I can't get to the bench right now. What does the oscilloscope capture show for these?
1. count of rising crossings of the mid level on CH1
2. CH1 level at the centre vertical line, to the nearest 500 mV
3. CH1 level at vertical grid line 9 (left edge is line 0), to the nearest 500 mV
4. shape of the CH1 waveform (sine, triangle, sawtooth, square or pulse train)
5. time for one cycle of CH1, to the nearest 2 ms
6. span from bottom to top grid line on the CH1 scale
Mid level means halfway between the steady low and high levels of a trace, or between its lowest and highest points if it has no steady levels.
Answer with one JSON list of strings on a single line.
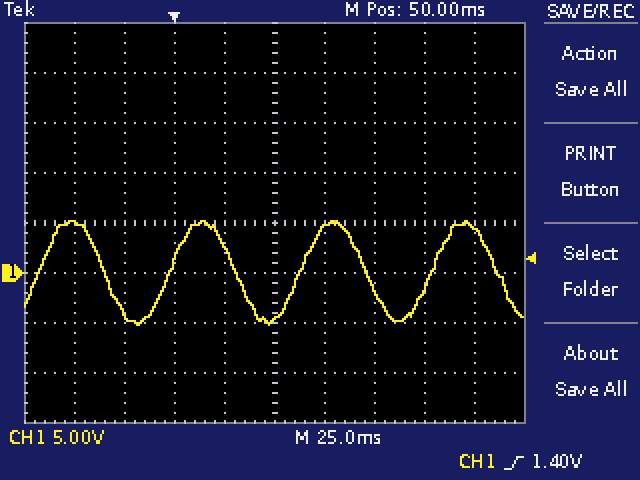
["4", "-4.5 V", "4.5 V", "sine", "66 ms", "40 V"]
